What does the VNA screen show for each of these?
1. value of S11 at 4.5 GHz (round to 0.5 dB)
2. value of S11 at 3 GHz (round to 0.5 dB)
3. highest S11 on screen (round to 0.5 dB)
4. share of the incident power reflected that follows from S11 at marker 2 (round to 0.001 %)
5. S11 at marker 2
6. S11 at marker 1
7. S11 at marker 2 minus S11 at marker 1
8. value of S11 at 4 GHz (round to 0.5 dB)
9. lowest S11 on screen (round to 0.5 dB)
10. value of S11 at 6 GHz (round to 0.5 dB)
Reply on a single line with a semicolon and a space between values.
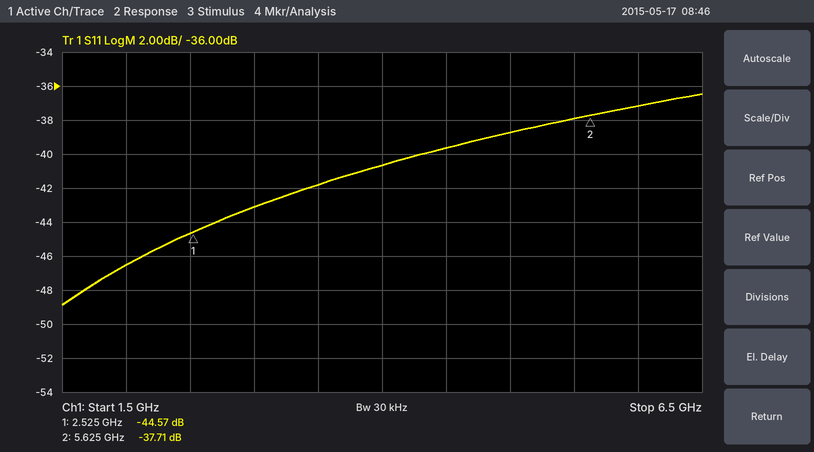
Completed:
-39.5 dB; -43.0 dB; -36.5 dB; 0.017 %; -37.71 dB; -44.57 dB; 6.86 dB; -40.5 dB; -49.0 dB; -37.0 dB
